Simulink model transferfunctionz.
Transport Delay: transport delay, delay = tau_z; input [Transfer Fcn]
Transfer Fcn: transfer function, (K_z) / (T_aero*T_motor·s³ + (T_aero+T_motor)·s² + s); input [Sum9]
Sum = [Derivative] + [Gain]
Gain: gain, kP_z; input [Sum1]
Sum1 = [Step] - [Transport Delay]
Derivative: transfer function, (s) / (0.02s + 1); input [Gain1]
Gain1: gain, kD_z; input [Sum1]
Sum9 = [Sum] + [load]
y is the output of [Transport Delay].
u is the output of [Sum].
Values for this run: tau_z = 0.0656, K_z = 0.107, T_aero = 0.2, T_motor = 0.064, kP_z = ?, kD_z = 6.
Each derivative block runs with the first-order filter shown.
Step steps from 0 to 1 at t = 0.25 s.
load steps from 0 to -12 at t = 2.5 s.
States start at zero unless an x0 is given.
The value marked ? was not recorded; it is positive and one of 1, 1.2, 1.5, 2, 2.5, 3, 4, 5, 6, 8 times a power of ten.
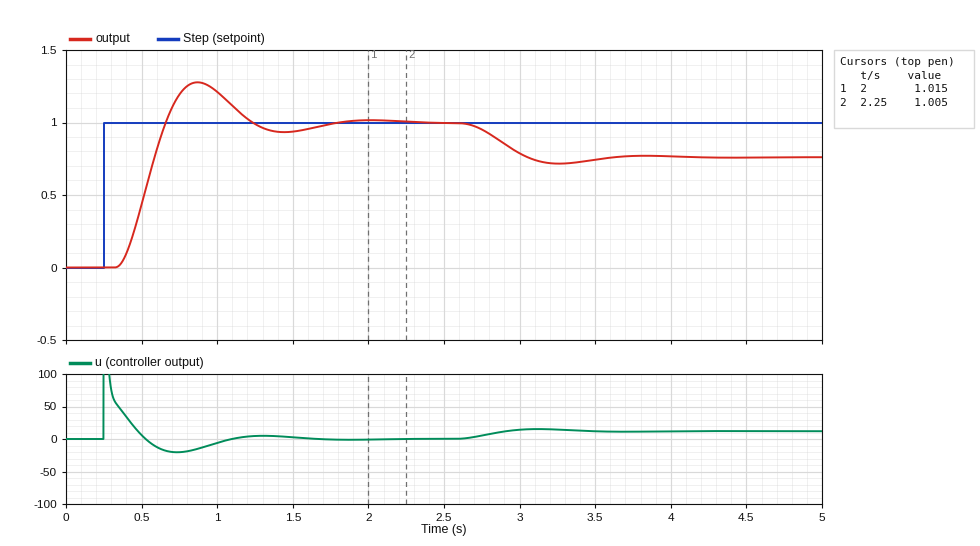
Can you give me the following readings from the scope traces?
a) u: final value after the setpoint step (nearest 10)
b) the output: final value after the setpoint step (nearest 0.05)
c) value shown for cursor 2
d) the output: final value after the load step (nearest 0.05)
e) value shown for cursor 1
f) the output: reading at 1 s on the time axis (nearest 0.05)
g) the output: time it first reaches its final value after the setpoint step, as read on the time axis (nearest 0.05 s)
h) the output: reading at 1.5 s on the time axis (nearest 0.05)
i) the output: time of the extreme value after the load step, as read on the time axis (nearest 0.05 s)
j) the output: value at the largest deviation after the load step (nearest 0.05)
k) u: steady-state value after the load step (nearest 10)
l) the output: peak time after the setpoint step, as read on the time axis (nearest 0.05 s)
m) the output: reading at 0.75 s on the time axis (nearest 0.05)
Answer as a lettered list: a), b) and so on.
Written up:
a) 0
b) 1.00
c) 1.005
d) 0.75
e) 1.015
f) 1.20
g) 0.65 s
h) 0.95
i) 3.25 s
j) 0.70
k) 10
l) 0.85 s
m) 1.20
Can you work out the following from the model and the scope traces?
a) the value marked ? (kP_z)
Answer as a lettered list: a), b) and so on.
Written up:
a) 50
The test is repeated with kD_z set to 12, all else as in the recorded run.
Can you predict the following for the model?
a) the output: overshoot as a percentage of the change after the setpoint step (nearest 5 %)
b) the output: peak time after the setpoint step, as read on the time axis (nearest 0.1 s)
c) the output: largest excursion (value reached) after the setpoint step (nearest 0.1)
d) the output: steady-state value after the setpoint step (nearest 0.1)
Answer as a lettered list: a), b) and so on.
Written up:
a) 25 %
b) 0.7 s
c) 1.2
d) 1.0
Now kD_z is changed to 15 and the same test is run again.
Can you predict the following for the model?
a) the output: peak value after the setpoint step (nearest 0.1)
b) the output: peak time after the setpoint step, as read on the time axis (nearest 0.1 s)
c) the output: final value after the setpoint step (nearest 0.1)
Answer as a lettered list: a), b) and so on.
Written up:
a) 1.3
b) 0.7 s
c) 1.0
